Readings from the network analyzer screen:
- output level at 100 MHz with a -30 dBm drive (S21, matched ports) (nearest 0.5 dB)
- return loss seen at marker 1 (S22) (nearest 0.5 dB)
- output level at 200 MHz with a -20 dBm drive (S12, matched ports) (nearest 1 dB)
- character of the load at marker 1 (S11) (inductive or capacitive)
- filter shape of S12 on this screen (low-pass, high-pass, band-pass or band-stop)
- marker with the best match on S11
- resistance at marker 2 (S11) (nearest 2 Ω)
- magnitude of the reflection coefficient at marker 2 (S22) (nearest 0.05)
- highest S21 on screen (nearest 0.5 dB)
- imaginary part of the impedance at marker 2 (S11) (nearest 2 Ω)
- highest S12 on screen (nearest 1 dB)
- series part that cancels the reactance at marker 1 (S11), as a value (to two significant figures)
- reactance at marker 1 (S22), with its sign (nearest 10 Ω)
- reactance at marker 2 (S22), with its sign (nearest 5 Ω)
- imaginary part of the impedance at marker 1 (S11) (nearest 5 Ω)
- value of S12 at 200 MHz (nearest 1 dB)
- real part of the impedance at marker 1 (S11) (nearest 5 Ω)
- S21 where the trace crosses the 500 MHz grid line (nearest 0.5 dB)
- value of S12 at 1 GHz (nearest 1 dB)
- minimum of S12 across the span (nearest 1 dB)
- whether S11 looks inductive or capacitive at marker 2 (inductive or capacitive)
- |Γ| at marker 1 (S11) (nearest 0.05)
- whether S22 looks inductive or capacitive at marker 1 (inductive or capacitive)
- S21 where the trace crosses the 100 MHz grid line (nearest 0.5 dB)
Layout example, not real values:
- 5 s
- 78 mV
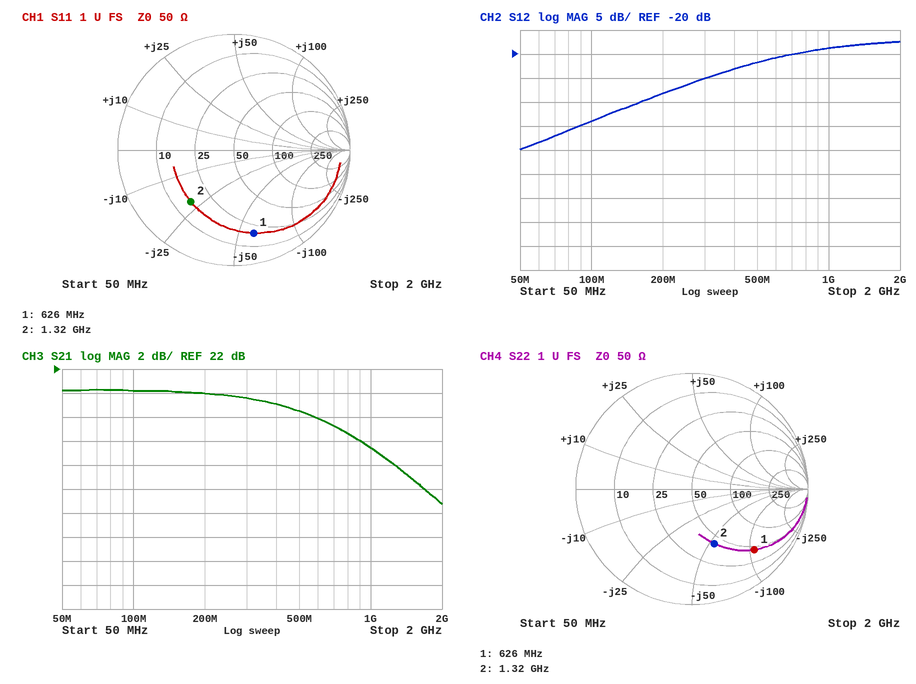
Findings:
- -10.0 dBm
- 2.5 dB
- -48 dBm
- capacitive
- high-pass
- marker 2
- 16 Ω
- 0.50
- 20.5 dB
- -22 Ω
- -17 dB
- 15 nH
- -110 Ω
- -55 Ω
- -60 Ω
- -28 dB
- 20 Ω
- 18.5 dB
- -19 dB
- -40 dB
- capacitive
- 0.75
- capacitive
- 20.0 dB
